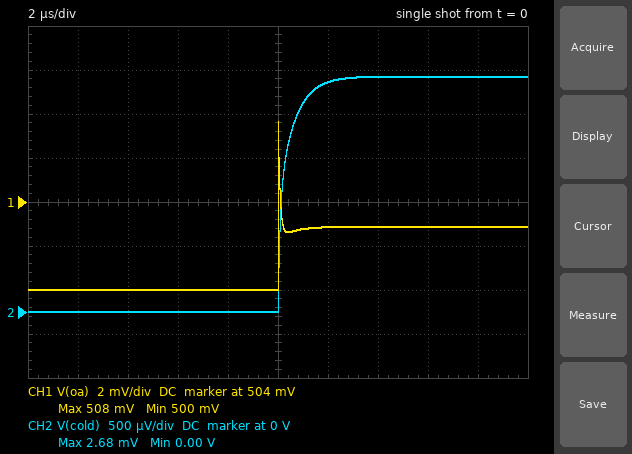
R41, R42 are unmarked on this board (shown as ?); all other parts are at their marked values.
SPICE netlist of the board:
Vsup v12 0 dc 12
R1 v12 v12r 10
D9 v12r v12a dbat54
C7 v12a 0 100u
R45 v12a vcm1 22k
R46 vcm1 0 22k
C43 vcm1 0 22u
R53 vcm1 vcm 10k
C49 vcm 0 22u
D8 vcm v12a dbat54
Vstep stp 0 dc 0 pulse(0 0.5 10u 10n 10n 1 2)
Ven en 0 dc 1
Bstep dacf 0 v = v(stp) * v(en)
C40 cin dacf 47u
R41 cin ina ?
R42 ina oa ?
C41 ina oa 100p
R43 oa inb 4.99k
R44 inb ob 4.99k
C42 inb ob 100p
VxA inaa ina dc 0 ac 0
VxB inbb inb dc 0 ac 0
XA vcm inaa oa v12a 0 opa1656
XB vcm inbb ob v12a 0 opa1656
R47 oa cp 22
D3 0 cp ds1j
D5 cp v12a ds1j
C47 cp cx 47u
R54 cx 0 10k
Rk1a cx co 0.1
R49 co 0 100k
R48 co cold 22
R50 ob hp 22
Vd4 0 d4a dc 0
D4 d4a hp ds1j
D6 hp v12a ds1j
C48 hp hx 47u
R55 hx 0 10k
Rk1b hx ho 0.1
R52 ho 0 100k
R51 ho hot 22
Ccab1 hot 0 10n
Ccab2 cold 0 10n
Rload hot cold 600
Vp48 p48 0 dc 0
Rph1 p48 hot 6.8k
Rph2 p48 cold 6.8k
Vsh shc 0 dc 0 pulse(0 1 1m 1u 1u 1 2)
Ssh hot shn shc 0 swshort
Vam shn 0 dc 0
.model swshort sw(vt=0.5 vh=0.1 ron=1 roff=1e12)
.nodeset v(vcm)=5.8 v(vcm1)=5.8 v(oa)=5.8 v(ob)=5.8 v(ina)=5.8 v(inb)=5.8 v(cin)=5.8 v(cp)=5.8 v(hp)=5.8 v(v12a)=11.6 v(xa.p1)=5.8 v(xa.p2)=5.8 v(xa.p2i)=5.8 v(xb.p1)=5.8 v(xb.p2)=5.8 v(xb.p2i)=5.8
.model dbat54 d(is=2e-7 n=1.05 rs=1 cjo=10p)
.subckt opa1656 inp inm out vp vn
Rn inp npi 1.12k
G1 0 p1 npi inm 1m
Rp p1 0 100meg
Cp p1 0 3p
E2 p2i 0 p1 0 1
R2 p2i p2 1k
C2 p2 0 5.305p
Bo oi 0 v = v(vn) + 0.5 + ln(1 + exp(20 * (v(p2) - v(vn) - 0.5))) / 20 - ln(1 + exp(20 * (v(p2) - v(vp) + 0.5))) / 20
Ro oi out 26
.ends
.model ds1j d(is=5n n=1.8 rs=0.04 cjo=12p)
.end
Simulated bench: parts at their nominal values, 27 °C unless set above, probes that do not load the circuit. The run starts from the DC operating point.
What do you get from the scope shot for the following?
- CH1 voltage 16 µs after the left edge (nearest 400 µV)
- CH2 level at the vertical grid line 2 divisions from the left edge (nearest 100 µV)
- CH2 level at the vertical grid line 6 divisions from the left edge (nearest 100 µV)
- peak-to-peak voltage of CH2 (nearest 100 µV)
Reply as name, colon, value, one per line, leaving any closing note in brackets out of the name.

CH1 voltage 16 µs after the left edge: 502.8 mV
CH2 level at the vertical grid line 2 divisions from the left edge: 0 V
CH2 level at the vertical grid line 6 divisions from the left edge: 2.6 mV
peak-to-peak voltage of CH2: 2.7 mV
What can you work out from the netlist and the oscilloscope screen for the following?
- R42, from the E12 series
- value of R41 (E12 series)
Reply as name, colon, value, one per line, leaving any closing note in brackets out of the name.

R42, from the E12 series: 3.3 kΩ
value of R41: 1 kΩ
